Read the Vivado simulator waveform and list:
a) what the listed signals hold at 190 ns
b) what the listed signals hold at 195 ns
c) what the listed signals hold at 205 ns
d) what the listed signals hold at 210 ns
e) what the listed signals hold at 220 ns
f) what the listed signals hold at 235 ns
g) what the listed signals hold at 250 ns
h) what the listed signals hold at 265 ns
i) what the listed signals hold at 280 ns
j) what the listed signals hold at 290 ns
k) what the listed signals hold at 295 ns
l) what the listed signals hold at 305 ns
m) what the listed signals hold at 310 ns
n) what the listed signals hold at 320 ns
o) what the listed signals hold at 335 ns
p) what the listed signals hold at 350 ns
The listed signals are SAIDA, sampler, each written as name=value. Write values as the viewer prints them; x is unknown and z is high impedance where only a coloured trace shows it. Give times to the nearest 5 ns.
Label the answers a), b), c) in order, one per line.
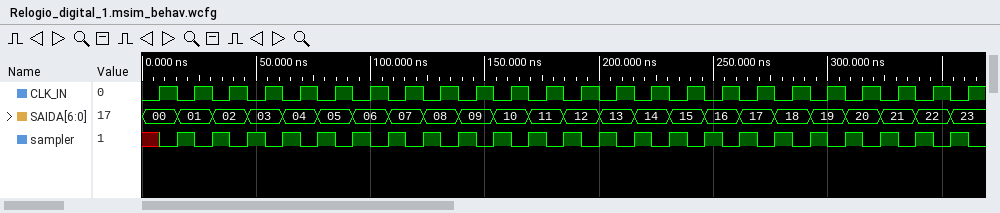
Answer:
a) SAIDA=12, sampler=1
b) SAIDA=12, sampler=0
c) SAIDA=13, sampler=1
d) SAIDA=13, sampler=0
e) SAIDA=14, sampler=1
f) SAIDA=15, sampler=1
g) SAIDA=16, sampler=1
h) SAIDA=17, sampler=1
i) SAIDA=18, sampler=1
j) SAIDA=18, sampler=0
k) SAIDA=19, sampler=1
l) SAIDA=19, sampler=0
m) SAIDA=20, sampler=1
n) SAIDA=20, sampler=0
o) SAIDA=21, sampler=0
p) SAIDA=22, sampler=0
